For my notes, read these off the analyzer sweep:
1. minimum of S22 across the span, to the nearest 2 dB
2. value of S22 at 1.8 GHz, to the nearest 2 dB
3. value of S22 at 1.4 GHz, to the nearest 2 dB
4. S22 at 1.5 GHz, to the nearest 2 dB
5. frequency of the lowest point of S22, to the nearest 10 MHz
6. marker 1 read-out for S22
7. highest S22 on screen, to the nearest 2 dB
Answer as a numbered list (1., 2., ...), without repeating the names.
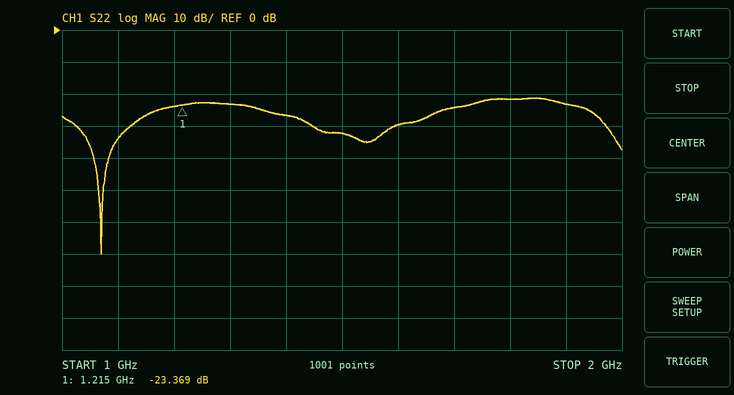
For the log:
1. -70 dB
2. -22 dB
3. -26 dB
4. -32 dB
5. 1.07 GHz
6. -23.369 dB
7. -22 dB
